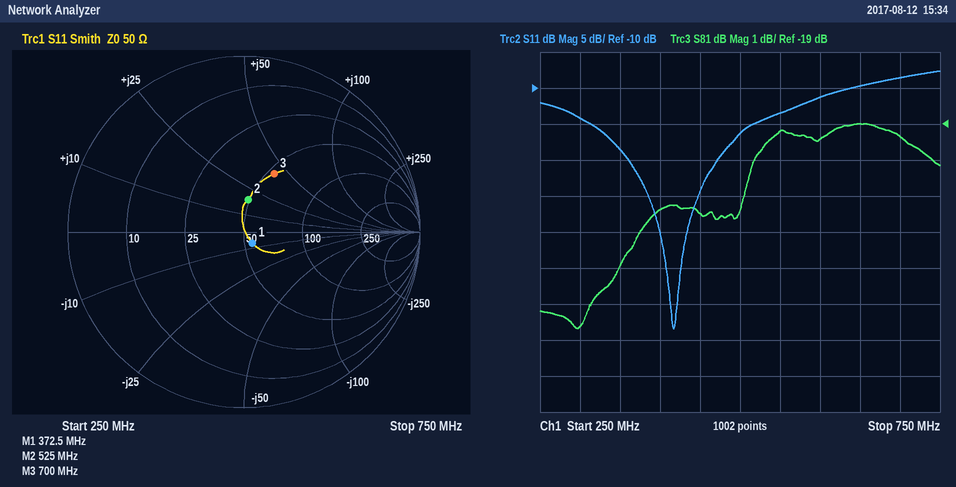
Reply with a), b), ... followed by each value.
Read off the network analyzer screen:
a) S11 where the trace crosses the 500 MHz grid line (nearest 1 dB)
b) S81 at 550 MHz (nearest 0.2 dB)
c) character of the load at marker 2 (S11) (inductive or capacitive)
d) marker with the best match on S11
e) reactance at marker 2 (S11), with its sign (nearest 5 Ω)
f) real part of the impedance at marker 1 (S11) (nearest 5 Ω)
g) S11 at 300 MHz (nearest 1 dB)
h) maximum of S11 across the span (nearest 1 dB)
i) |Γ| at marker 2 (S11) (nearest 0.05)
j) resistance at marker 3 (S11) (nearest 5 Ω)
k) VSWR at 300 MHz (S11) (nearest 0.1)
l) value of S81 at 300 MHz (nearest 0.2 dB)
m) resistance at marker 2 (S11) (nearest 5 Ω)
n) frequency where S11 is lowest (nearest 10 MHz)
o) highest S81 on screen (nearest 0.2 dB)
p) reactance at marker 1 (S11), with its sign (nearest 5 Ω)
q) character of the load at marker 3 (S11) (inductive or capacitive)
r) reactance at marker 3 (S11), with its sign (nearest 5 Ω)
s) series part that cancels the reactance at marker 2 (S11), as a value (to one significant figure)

a) -16 dB
b) -19.2 dB
c) inductive
d) marker 1
e) +20 Ω
f) 55 Ω
g) -14 dB
h) -8 dB
i) 0.20
j) 55 Ω
k) 1.5
l) -24.6 dB
m) 50 Ω
n) 420 MHz
o) -19.0 dB
p) -5 Ω
q) inductive
r) +40 Ω
s) 20 pF
